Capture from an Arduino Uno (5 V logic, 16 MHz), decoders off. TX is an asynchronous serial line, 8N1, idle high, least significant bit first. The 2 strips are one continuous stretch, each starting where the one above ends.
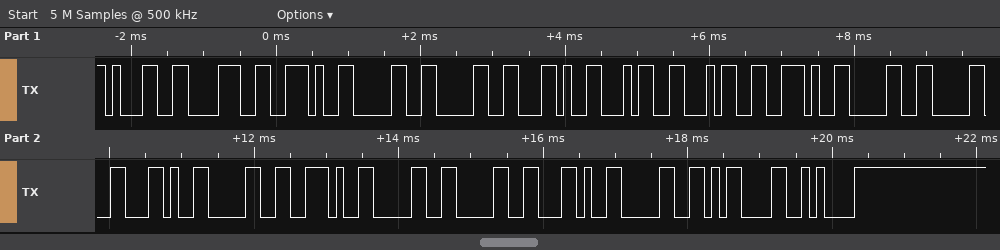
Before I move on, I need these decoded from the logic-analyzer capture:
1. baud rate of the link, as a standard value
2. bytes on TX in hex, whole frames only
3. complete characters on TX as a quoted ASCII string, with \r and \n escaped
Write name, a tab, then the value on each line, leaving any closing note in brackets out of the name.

baud rate of the link, as a standard value	9600 baud
bytes on TX in hex, whole frames only	31 38 2E 30 30 2C 34 34 2E 30 30 2C 30 2E 30 30 2C 30 0D 0A
complete characters on TX as a quoted ASCII string, with \r and \n escaped	"18.00,44.00,0.00,0\r\n"
